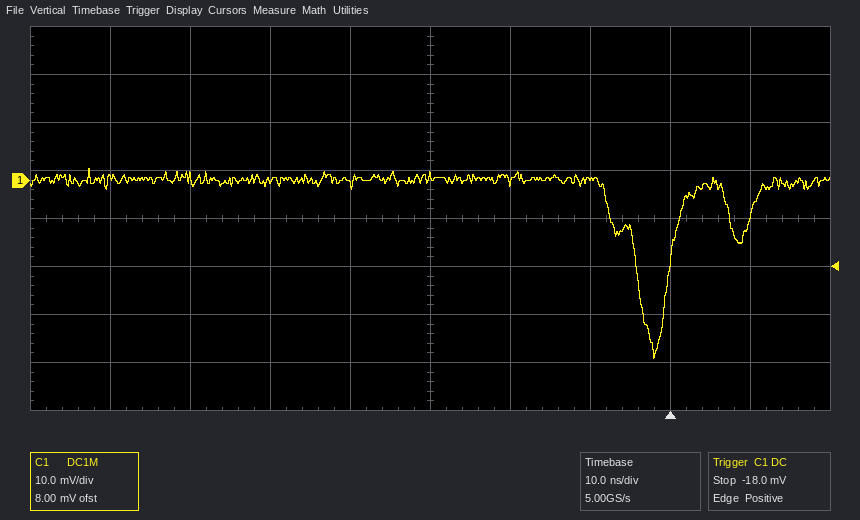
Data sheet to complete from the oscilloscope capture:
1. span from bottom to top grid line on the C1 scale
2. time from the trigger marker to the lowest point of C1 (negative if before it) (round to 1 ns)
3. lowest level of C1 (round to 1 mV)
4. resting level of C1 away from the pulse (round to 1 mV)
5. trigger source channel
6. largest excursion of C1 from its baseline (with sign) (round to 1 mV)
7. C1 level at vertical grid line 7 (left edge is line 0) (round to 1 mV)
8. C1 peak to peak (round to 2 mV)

80 mV
-2 ns
-37 mV
0 mV
C1
-37 mV
0 mV
40 mV
